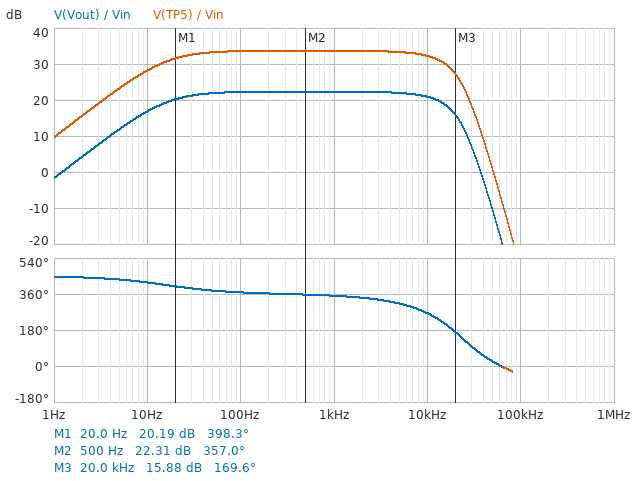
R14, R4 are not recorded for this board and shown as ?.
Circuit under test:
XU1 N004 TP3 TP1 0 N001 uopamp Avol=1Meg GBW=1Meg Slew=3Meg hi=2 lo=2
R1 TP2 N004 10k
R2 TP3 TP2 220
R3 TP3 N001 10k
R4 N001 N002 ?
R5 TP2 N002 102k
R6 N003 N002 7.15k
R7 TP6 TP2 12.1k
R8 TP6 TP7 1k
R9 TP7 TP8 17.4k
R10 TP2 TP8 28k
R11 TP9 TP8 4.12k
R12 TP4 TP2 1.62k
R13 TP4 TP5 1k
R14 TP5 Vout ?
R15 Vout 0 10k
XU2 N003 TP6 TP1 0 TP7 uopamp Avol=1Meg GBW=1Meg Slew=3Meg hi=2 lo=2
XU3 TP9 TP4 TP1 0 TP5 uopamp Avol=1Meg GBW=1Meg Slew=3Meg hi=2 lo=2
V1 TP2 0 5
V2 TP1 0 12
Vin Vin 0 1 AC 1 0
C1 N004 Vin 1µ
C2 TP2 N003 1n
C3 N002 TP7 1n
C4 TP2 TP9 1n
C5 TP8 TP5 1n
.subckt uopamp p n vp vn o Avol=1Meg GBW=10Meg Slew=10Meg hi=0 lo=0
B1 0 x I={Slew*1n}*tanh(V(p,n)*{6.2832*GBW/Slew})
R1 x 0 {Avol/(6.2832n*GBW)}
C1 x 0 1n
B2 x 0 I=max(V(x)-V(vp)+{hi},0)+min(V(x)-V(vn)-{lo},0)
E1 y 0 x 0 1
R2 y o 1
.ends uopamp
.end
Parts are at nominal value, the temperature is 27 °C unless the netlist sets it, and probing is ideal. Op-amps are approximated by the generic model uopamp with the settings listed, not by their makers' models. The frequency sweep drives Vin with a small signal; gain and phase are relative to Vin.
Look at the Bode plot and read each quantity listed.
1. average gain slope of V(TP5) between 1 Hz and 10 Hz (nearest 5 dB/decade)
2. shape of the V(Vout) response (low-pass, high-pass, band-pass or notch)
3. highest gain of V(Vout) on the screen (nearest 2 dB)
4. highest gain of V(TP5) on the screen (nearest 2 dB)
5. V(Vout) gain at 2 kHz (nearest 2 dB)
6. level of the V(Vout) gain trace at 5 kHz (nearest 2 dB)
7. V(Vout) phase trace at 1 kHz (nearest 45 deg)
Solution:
20 dB/decade
band-pass
22 dB
34 dB
22 dB
22 dB
360 deg
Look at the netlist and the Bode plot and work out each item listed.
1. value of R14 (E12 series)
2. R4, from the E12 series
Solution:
27 kΩ
3.9 kΩ
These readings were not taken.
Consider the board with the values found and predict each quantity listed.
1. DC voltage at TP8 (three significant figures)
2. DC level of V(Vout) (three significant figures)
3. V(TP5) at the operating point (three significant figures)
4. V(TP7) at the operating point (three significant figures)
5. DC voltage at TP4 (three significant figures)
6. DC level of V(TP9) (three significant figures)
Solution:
5.00 V
1.35 V
5.00 V
5.00 V
5.00 V
5.00 V
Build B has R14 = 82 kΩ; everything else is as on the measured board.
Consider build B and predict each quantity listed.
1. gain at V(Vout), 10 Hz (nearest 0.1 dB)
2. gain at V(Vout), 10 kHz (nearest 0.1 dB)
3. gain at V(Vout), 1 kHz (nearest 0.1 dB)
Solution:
8.9 dB
13.0 dB
14.4 dB
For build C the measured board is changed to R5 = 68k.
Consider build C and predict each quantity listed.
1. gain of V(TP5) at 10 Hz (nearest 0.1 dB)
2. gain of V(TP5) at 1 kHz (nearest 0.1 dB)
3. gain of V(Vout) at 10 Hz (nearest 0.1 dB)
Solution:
28.0 dB
33.5 dB
16.7 dB
